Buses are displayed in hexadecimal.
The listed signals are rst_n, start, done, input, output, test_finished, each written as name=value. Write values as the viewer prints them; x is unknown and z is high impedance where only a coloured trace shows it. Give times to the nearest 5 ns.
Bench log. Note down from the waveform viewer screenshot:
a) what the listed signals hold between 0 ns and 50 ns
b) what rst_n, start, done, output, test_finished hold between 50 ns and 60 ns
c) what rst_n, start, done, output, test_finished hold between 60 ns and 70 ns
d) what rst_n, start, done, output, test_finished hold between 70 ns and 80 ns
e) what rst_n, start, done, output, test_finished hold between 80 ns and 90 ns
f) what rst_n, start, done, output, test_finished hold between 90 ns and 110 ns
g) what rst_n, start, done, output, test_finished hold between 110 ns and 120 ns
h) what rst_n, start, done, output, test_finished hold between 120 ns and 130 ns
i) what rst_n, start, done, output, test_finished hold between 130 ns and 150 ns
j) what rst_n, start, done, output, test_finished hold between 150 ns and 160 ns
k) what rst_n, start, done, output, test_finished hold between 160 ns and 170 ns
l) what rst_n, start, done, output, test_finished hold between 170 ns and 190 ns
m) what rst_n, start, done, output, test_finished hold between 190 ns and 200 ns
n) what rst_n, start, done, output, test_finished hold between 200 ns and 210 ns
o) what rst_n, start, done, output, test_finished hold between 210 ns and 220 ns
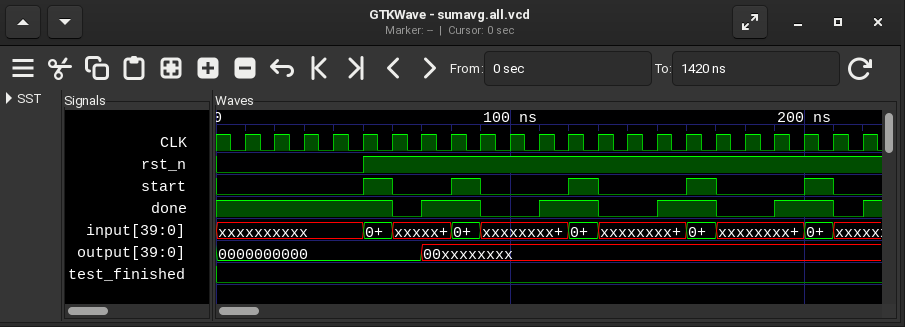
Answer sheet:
rst_n=0, start=0, done=1, input=xxxxxxxxxx, output=0000000000, test_finished=0
rst_n=1, start=1, done=1, output=0000000000, test_finished=0
rst_n=1, start=0, done=0, output=0000000000, test_finished=0
rst_n=1, start=0, done=1, output=00xxxxxxxx, test_finished=0
rst_n=1, start=1, done=1, output=00xxxxxxxx, test_finished=0
rst_n=1, start=0, done=0, output=00xxxxxxxx, test_finished=0
rst_n=1, start=0, done=1, output=00xxxxxxxx, test_finished=0
rst_n=1, start=1, done=1, output=00xxxxxxxx, test_finished=0
rst_n=1, start=0, done=0, output=00xxxxxxxx, test_finished=0
rst_n=1, start=0, done=1, output=00xxxxxxxx, test_finished=0
rst_n=1, start=1, done=1, output=00xxxxxxxx, test_finished=0
rst_n=1, start=0, done=0, output=00xxxxxxxx, test_finished=0
rst_n=1, start=0, done=1, output=00xxxxxxxx, test_finished=0
rst_n=1, start=1, done=1, output=00xxxxxxxx, test_finished=0
rst_n=1, start=0, done=0, output=00xxxxxxxx, test_finished=0
